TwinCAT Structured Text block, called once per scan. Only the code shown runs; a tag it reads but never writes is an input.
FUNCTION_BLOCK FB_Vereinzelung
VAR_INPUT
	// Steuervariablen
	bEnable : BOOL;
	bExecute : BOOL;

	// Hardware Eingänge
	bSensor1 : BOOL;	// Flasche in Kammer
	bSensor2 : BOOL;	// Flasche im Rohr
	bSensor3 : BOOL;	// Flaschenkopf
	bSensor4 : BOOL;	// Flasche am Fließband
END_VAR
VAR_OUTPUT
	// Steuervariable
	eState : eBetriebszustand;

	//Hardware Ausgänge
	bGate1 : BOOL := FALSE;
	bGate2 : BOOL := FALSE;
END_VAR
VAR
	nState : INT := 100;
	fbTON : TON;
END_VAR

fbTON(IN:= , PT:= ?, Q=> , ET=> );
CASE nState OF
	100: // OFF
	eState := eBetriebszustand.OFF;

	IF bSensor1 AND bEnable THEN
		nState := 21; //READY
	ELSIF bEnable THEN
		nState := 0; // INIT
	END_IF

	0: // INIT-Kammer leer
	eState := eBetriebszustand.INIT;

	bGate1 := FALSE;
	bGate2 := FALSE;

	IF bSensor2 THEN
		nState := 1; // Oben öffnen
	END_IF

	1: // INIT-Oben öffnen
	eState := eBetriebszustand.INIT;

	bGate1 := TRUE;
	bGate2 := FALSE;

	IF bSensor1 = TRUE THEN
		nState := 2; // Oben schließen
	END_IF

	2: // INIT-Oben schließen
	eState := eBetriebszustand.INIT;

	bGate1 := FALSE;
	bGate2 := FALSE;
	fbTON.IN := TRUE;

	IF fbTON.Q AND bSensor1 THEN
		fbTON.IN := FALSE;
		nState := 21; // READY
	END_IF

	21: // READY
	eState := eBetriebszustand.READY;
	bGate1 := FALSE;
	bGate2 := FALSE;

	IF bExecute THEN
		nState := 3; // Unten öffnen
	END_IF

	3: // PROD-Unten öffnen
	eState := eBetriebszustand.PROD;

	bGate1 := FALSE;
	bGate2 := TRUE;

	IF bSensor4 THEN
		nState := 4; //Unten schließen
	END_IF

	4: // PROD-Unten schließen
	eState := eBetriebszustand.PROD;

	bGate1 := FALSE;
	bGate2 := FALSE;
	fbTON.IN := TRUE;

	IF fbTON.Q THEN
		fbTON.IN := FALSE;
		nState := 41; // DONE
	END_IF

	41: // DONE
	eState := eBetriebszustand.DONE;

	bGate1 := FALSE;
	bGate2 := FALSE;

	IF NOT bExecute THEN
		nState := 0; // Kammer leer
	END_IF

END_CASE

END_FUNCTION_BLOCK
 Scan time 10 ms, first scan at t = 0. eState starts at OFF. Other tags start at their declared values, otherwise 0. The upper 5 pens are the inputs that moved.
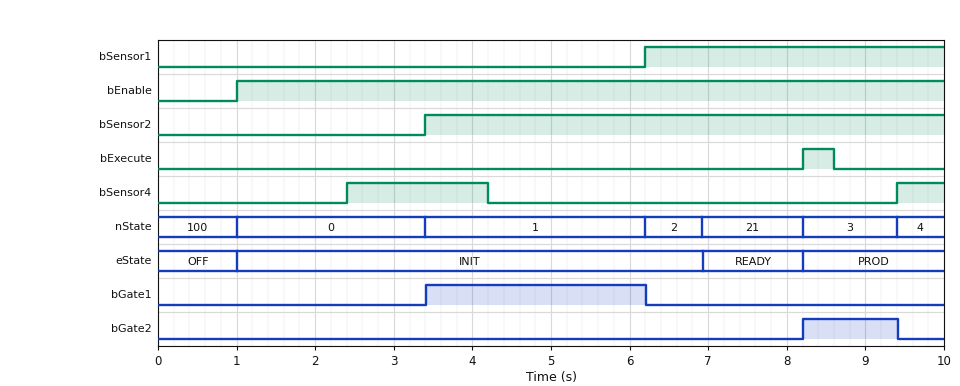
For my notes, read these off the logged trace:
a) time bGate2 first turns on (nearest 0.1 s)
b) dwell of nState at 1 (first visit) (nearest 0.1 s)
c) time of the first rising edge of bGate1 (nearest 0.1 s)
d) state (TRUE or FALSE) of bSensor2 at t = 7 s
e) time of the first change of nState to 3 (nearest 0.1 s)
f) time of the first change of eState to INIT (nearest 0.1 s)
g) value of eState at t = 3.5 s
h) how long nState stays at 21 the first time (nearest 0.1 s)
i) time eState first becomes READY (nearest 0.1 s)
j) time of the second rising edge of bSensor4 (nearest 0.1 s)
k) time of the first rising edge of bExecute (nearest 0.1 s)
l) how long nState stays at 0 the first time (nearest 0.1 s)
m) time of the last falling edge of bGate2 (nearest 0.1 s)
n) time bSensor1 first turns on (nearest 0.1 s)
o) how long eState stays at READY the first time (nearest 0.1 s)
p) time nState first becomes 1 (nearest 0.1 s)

8.2 s
2.8 s
3.4 s
TRUE
8.2 s
1.0 s
INIT
1.3 s
6.9 s
9.4 s
8.2 s
2.4 s
9.4 s
6.2 s
1.3 s
3.4 s
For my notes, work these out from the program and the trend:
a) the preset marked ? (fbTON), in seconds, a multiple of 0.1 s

0.7 s
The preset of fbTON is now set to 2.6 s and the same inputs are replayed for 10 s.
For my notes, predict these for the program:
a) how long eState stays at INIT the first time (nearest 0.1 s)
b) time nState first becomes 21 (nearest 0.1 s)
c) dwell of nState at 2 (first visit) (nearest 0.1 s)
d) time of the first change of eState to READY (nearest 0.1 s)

7.8 s
8.8 s
2.6 s
8.8 s
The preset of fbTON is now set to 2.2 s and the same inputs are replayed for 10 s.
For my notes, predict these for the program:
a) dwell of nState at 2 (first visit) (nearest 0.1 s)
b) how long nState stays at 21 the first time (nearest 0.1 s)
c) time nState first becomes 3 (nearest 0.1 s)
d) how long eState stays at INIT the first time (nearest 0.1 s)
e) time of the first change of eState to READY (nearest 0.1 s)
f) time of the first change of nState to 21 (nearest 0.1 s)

2.2 s
0.0 s
8.4 s
7.4 s
8.4 s
8.4 s
